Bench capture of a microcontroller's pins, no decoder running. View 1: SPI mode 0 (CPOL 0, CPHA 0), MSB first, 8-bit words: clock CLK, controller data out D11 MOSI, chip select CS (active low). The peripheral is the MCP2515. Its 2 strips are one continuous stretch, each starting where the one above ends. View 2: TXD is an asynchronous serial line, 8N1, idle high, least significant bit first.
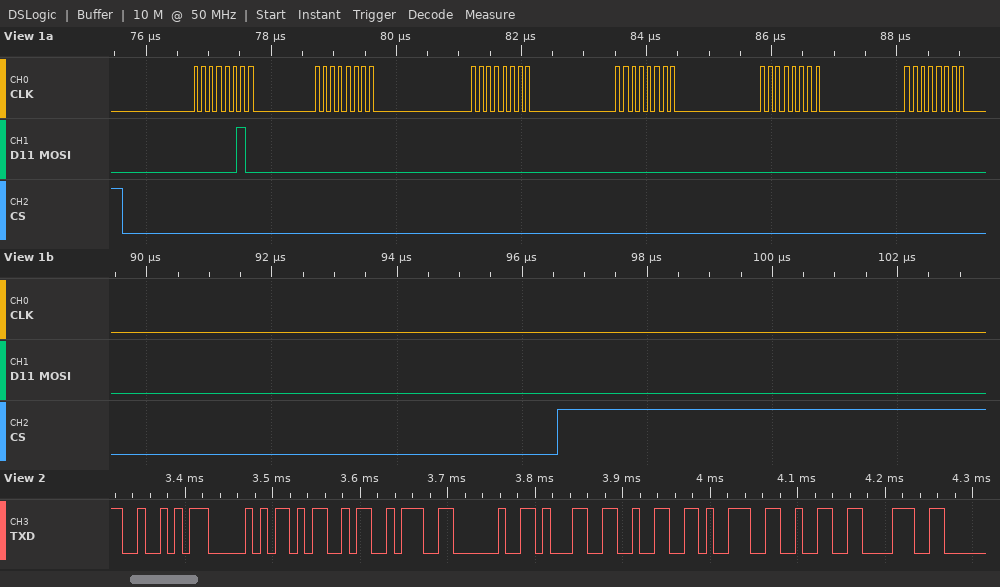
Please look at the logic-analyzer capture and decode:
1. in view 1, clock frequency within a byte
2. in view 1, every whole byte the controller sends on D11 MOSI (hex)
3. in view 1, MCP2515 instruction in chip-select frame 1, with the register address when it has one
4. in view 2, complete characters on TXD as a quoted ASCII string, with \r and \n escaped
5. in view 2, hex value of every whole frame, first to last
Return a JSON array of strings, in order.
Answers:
["8 MHz", "0x02 0x00 0x00 0x00 0x00 0x00", "WRITE 0x00", "\"RPM: 12928\"", "52 50 4D 3A 20 31 32 39 32 38"]
